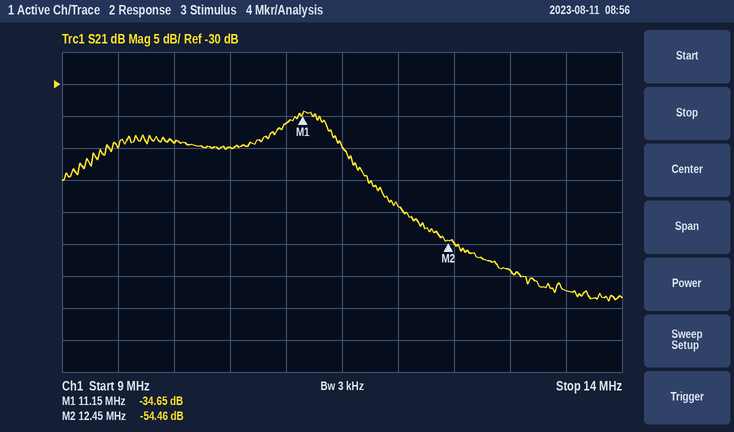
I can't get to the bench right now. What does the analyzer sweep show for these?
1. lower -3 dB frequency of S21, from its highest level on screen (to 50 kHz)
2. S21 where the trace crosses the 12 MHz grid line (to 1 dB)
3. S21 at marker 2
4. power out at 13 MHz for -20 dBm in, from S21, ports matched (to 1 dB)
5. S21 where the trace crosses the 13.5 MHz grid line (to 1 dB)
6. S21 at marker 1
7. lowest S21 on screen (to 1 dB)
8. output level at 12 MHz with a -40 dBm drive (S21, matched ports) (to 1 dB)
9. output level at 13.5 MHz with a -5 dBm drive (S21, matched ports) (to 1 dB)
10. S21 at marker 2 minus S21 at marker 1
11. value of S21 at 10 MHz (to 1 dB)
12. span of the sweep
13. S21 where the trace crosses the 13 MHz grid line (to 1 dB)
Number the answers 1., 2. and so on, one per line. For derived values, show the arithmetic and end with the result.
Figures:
1. 10.90 MHz
2. -49 dB
3. -54.46 dB
4. -20 dBm + (-59 dB) = -79 dBm
5. -62 dB
6. -34.65 dB
7. -64 dB
8. -40 dBm + (-49 dB) = -89 dBm
9. -5 dBm + (-62 dB) = -67 dBm
10. -54.46 − (-34.65) = -19.81 dB
11. -39 dB
12. 5 MHz
13. -59 dB
